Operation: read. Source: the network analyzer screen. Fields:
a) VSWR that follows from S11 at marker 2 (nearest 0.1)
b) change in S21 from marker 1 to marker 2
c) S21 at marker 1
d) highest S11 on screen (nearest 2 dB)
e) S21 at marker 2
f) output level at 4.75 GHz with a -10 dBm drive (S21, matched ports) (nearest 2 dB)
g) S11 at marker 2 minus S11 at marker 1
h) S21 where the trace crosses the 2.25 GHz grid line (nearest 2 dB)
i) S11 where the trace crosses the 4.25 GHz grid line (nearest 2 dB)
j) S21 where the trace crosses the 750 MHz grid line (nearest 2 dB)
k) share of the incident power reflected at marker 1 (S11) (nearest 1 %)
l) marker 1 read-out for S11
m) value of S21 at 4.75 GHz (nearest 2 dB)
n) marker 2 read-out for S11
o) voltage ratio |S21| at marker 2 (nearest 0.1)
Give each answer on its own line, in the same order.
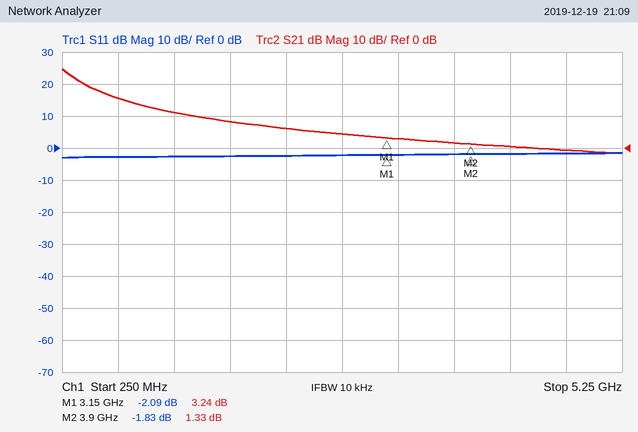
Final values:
9.5
-1.91 dB
3.24 dB
-2 dB
1.33 dB
-10 dBm
0.26 dB
6 dB
-2 dB
16 dB
62 %
-2.09 dB
0 dB
-1.83 dB
1.2
